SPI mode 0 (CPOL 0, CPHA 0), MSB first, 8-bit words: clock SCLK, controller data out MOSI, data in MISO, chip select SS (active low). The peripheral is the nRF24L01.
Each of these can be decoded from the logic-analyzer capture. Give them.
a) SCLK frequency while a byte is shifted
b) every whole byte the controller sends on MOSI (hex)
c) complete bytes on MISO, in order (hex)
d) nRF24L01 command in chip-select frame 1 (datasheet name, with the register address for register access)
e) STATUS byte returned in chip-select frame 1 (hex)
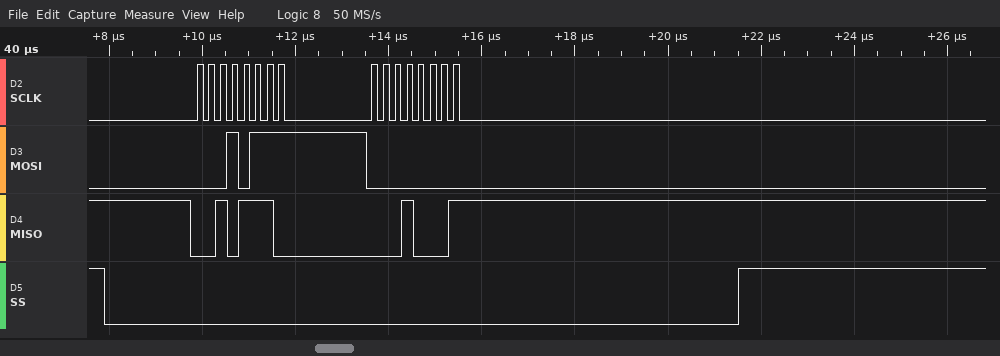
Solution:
4 MHz
17 00
2E 11
R_REGISTER 0x17
0x2E
